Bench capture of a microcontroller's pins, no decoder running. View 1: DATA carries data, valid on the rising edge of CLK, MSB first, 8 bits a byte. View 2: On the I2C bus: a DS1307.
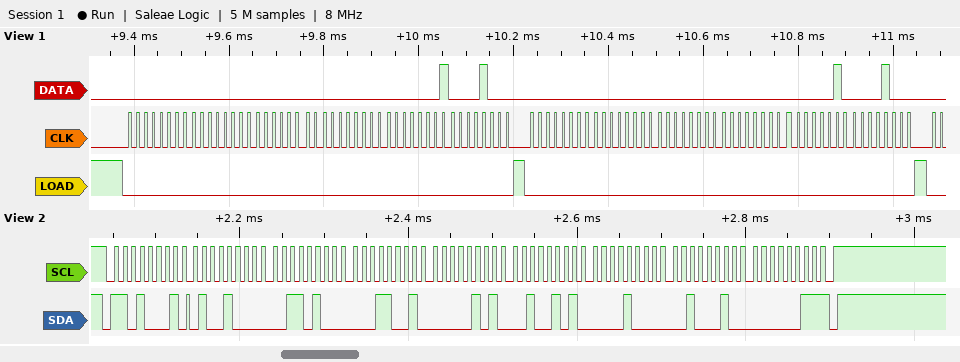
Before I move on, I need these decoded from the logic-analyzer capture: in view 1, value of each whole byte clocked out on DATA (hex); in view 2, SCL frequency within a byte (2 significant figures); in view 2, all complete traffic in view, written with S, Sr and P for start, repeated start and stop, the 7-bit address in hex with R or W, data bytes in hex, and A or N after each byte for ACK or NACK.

00 00 00 00 01 08 00 00 00 00 02 08
100 kHz
S 68R A 48 A 34 A 19 A 05 A 25 A 08 A 22 A 03 N P
